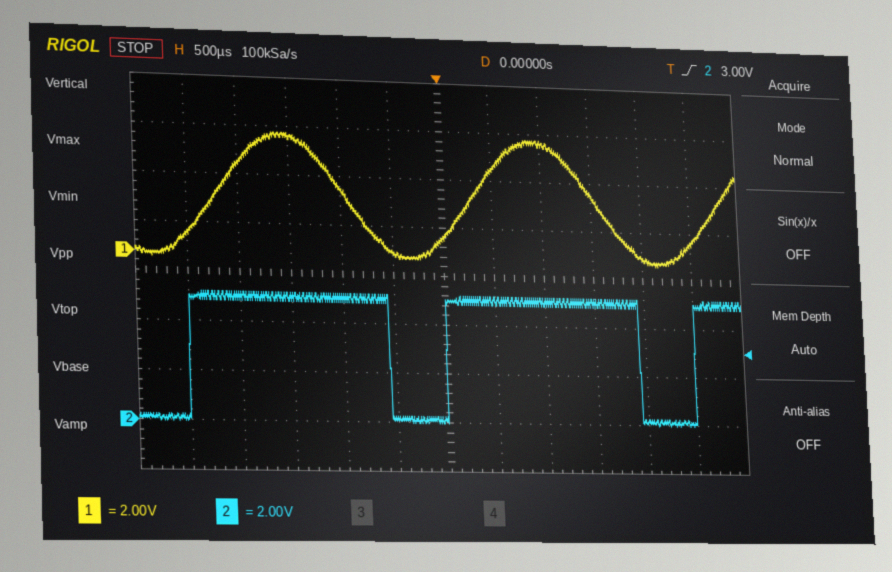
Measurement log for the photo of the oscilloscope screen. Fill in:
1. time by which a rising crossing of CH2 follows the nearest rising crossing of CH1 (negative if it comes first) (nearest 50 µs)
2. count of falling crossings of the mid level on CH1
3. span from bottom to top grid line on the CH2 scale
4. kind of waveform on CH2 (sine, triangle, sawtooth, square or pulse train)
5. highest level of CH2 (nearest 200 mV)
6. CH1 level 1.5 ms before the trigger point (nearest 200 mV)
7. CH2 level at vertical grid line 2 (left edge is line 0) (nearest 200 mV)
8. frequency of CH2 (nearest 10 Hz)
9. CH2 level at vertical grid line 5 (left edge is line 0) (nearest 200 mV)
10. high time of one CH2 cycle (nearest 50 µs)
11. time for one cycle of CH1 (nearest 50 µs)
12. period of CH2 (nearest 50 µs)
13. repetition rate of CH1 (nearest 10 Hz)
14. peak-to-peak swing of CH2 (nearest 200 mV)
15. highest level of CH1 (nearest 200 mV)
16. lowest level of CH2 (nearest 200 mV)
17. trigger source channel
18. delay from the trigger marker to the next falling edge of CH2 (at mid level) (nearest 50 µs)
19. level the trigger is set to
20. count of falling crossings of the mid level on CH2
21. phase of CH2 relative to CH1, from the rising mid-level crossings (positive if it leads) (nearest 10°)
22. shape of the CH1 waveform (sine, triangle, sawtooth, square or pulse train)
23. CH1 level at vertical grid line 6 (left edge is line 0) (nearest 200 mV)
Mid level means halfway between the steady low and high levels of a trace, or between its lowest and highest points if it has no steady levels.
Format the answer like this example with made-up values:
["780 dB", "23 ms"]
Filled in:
["-300 µs", "2", "16 V", "pulse train", "5.2 V", "4.8 V", "5.0 V", "400 Hz", "200 mV", "1.95 ms", "2.50 ms", "2.50 ms", "400 Hz", "5.2 V", "5.0 V", "0.0 V", "CH2", "1.95 ms", "3.00 V", "2", "+40°", "sine", "800 mV"]
